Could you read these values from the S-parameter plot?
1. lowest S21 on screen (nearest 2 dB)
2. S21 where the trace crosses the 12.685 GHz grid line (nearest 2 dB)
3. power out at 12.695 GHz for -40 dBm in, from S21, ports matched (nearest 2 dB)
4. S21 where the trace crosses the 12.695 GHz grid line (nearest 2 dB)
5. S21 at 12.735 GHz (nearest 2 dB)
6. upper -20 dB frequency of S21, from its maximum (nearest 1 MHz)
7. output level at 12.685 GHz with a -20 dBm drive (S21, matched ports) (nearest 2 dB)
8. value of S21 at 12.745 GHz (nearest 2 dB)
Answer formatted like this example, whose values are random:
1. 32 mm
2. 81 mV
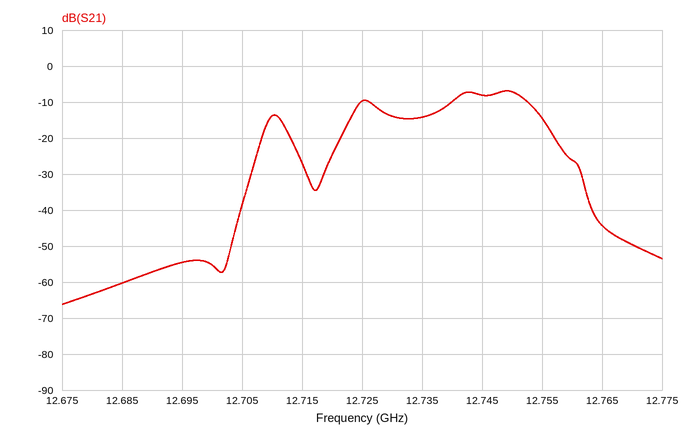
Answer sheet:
1. -66 dB
2. -60 dB
3. -94 dBm
4. -54 dB
5. -14 dB
6. 12.761 GHz
7. -80 dBm
8. -8 dB
